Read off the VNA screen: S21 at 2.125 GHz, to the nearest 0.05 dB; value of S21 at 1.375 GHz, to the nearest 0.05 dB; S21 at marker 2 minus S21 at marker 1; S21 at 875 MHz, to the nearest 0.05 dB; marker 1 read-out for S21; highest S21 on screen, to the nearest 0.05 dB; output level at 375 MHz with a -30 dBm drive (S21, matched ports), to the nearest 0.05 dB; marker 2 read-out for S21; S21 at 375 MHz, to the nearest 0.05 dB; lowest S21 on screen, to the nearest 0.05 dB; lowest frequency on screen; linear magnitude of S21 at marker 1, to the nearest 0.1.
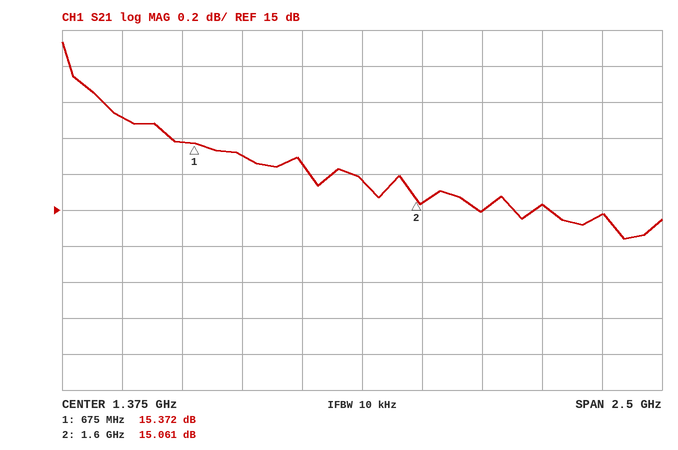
15.05 dB
15.15 dB
-0.311 dB
15.30 dB
15.372 dB
15.95 dB
-14.50 dBm
15.061 dB
15.50 dB
14.85 dB
125 MHz
5.9
